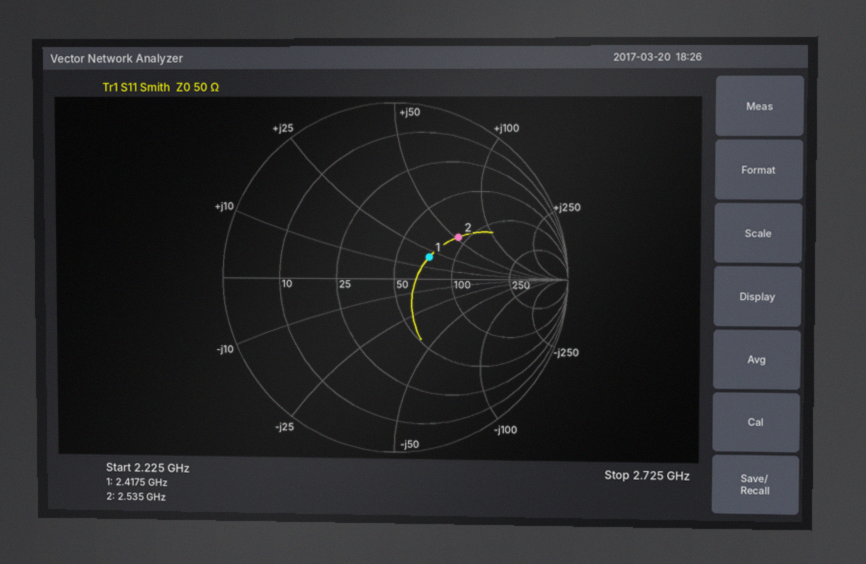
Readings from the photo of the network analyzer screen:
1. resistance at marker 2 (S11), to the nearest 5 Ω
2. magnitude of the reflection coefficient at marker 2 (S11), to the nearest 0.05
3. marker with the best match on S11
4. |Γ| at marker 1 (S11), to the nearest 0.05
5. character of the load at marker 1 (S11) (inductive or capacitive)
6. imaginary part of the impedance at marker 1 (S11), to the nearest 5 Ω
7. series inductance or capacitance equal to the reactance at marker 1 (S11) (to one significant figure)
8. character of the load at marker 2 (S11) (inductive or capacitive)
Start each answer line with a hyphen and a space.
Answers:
- 90 Ω
- 0.45
- marker 1
- 0.25
- inductive
- +20 Ω
- 1 nH
- inductive
